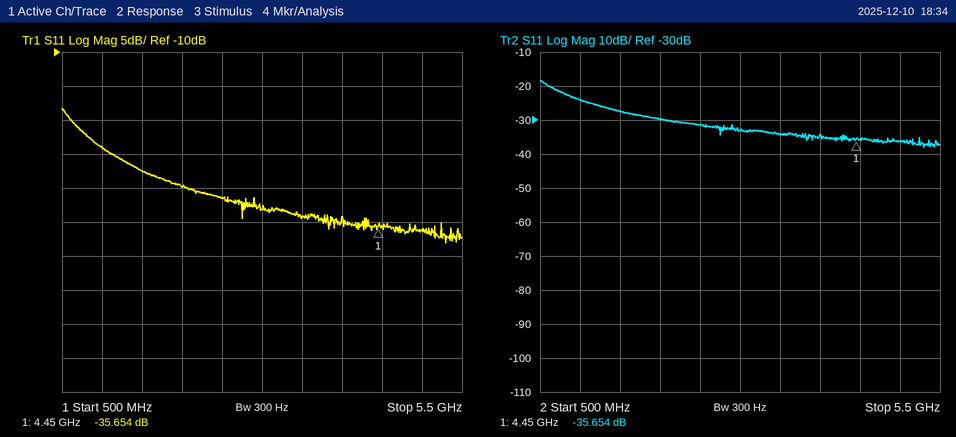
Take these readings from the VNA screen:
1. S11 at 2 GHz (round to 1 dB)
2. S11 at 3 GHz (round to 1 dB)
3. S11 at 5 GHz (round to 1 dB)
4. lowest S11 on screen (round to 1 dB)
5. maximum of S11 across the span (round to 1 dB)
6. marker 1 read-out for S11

-30 dB
-33 dB
-36 dB
-38 dB
-18 dB
-35.654 dB
